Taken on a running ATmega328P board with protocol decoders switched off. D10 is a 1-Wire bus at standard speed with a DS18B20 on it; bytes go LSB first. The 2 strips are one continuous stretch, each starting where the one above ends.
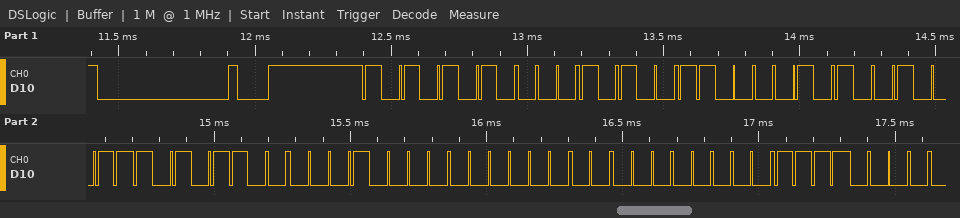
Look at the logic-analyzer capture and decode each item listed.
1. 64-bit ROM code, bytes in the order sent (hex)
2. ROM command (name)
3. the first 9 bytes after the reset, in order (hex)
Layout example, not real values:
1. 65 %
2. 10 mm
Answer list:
1. 28 43 C9 35 08 00 00 0F
2. Match ROM
3. 55 28 43 C9 35 08 00 00 0F
